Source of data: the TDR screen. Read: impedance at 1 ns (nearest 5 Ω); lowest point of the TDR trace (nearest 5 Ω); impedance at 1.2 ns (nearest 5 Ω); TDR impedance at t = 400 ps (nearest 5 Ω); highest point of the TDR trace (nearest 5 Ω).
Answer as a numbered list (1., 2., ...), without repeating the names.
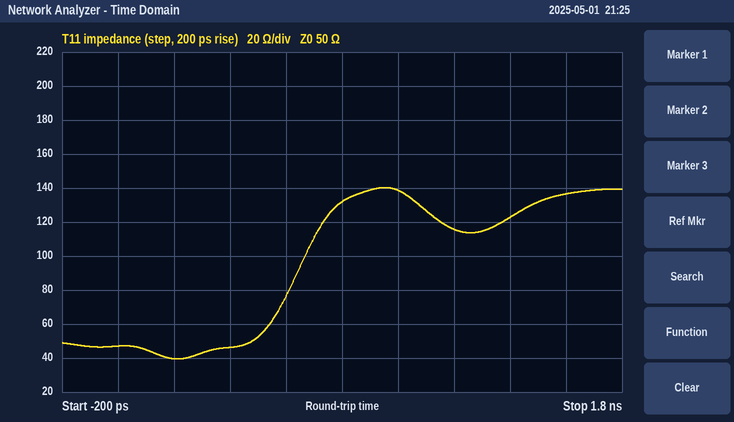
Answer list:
1. 140 Ω
2. 40 Ω
3. 115 Ω
4. 45 Ω
5. 140 Ω
